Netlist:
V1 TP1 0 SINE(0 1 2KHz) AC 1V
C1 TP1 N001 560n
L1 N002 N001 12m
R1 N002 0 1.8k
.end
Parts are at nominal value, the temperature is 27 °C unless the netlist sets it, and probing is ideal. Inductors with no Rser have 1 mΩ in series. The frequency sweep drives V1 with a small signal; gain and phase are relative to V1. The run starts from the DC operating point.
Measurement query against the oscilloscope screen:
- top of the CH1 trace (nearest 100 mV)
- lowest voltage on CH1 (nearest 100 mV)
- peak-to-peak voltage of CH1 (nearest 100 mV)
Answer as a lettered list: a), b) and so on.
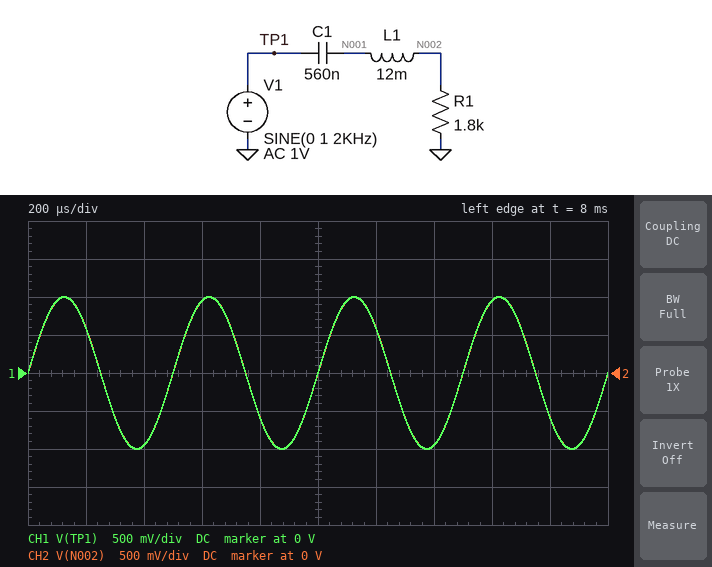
a) 1.0 V
b) -1.0 V
c) 2.0 V
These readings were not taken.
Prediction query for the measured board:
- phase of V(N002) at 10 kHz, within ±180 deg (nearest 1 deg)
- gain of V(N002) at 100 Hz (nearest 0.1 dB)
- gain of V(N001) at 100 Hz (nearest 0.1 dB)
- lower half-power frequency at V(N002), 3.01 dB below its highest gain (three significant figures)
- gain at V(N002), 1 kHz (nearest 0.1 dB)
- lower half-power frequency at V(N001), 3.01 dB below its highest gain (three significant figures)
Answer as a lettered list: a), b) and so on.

a) -22 deg
b) -5.4 dB
c) -5.4 dB
d) 157 Hz
e) -0.1 dB
f) 159 Hz
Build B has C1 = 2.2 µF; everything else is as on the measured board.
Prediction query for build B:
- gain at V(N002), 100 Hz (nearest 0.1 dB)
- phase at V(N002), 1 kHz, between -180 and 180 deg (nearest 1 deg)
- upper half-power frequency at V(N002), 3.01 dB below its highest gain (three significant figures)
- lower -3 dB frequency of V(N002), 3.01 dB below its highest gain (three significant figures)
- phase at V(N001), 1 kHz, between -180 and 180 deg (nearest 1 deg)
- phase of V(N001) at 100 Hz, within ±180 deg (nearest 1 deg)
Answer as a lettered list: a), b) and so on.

a) -0.6 dB
b) 0 deg
c) 23.9 kHz
d) 40.1 Hz
e) 2 deg
f) 22 deg
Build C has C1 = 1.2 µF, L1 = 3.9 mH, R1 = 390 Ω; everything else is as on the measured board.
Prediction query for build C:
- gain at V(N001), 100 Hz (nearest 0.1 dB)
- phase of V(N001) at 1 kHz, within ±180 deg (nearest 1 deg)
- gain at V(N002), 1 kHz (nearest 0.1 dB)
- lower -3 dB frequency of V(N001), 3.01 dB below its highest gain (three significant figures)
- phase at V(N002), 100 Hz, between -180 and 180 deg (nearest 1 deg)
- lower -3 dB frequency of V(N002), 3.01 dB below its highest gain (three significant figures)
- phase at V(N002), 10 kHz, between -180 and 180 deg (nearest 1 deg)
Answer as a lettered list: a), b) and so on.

a) -11.0 dB
b) 19 deg
c) -0.3 dB
d) 345 Hz
e) 74 deg
f) 333 Hz
g) -31 deg
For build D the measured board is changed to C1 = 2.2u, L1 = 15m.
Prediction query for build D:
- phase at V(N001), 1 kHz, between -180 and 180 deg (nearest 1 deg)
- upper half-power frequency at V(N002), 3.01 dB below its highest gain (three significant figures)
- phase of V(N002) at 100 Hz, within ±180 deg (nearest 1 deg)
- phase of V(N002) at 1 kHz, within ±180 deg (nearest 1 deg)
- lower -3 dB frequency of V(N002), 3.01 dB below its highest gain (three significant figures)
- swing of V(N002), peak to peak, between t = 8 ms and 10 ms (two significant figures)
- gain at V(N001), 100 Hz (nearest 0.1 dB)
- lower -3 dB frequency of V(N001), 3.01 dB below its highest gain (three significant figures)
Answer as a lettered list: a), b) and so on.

a) 2 deg
b) 19.1 kHz
c) 22 deg
d) -1 deg
e) 40.1 Hz
f) 2.0 V
g) -0.6 dB
h) 40.3 Hz
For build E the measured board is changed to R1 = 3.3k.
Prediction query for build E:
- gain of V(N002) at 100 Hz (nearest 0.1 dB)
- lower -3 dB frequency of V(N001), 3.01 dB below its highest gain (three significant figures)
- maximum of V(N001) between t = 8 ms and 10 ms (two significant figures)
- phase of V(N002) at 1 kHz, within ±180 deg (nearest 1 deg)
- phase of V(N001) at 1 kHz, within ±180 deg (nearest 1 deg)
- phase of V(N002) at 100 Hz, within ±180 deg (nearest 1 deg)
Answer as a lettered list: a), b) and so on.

a) -2.4 dB
b) 86.3 Hz
c) 1.0 V
d) 4 deg
e) 5 deg
f) 41 deg
